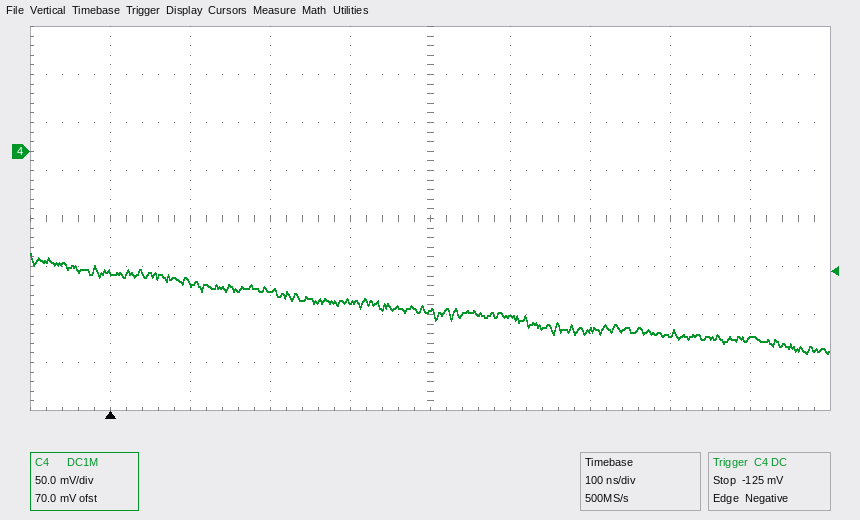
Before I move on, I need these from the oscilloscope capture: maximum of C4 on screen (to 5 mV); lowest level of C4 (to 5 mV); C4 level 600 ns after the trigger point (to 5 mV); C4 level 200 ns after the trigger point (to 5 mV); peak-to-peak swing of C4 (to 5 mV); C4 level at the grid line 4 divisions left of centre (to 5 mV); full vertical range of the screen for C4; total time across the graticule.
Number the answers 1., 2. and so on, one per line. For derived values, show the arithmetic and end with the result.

1. -105 mV
2. -210 mV
3. -185 mV
4. -145 mV
5. -105 mV − (-210 mV) = 105 mV
6. -125 mV
7. 400 mV
8. 1 µs
